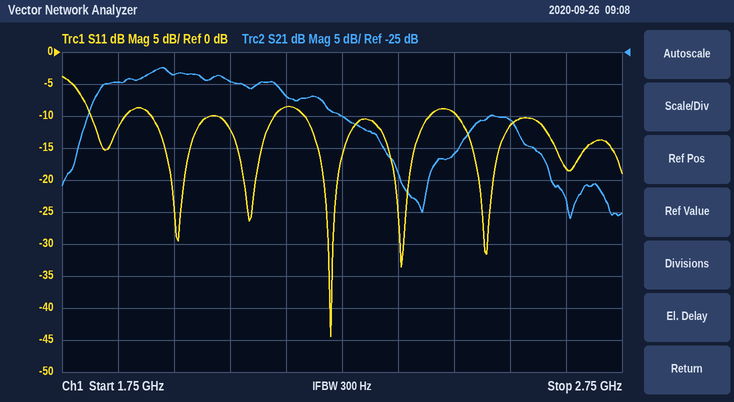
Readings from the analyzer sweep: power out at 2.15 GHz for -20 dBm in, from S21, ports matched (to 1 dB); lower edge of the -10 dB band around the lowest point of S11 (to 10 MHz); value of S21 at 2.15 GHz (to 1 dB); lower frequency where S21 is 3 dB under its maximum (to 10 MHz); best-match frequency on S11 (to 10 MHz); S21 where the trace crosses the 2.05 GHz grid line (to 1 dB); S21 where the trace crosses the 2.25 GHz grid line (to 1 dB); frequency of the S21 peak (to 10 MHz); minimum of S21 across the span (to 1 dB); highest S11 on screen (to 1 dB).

-52 dBm
2.18 GHz
-32 dB
1.82 GHz
2.23 GHz
-30 dB
-35 dB
1.93 GHz
-51 dB
-4 dB
